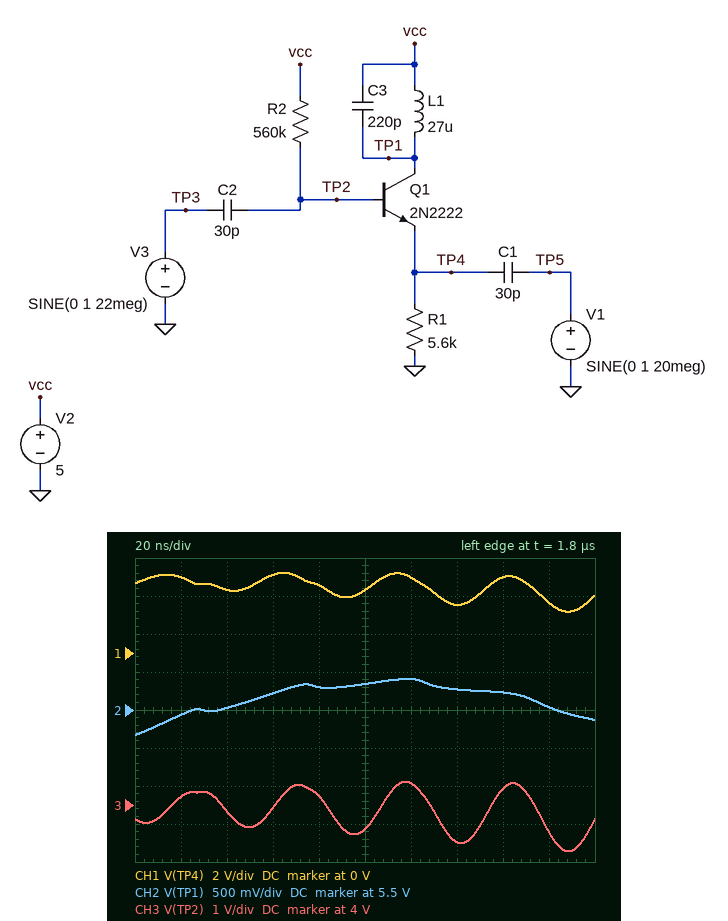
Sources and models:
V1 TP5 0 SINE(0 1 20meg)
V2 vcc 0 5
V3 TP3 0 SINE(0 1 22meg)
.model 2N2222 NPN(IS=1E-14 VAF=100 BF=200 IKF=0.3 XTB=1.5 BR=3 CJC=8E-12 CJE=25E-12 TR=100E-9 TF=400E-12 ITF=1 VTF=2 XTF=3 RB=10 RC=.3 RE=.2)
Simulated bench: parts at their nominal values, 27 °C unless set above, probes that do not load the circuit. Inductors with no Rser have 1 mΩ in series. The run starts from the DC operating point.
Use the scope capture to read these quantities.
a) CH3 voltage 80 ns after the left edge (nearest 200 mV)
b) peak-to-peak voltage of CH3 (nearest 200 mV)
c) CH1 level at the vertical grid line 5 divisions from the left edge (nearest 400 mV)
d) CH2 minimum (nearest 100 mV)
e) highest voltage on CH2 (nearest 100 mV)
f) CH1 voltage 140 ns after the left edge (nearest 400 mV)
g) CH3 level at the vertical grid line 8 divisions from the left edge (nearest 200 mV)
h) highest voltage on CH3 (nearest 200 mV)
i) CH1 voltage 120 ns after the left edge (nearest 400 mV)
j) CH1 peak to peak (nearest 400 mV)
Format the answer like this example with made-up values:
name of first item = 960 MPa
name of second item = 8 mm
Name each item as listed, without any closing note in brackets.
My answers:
CH3 voltage 80 ns after the left edge = 4.2 V
peak-to-peak voltage of CH3 = 1.8 V
CH1 level at the vertical grid line 5 divisions from the left edge = 3.2 V
CH2 minimum = 5.2 V
highest voltage on CH2 = 5.9 V
CH1 voltage 140 ns after the left edge = 2.4 V
CH3 level at the vertical grid line 8 divisions from the left edge = 4.4 V
highest voltage on CH3 = 4.6 V
CH1 voltage 120 ns after the left edge = 4.0 V
CH1 peak to peak = 2.0 V
